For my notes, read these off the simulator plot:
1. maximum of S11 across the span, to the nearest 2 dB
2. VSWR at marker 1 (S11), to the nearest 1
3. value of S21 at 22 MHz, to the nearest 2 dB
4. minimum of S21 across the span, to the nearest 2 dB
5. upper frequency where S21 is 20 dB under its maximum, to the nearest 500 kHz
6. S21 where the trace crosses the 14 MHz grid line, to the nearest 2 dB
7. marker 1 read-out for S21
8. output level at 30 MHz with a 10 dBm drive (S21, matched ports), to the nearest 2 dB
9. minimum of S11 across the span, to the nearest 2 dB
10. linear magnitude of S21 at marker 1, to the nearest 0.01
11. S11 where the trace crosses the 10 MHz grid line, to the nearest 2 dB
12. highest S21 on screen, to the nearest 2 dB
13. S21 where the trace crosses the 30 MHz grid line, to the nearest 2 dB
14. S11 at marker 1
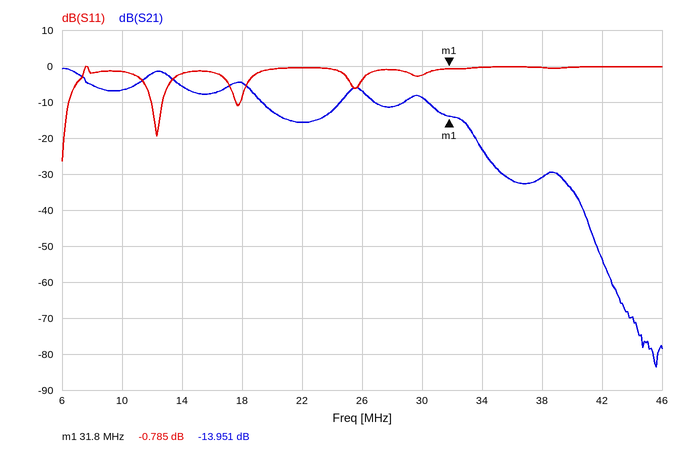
0 dB
22
-16 dB
-84 dB
33.5 MHz
-6 dB
-13.951 dB
2 dBm
-26 dB
0.20
-2 dB
0 dB
-8 dB
-0.785 dB
